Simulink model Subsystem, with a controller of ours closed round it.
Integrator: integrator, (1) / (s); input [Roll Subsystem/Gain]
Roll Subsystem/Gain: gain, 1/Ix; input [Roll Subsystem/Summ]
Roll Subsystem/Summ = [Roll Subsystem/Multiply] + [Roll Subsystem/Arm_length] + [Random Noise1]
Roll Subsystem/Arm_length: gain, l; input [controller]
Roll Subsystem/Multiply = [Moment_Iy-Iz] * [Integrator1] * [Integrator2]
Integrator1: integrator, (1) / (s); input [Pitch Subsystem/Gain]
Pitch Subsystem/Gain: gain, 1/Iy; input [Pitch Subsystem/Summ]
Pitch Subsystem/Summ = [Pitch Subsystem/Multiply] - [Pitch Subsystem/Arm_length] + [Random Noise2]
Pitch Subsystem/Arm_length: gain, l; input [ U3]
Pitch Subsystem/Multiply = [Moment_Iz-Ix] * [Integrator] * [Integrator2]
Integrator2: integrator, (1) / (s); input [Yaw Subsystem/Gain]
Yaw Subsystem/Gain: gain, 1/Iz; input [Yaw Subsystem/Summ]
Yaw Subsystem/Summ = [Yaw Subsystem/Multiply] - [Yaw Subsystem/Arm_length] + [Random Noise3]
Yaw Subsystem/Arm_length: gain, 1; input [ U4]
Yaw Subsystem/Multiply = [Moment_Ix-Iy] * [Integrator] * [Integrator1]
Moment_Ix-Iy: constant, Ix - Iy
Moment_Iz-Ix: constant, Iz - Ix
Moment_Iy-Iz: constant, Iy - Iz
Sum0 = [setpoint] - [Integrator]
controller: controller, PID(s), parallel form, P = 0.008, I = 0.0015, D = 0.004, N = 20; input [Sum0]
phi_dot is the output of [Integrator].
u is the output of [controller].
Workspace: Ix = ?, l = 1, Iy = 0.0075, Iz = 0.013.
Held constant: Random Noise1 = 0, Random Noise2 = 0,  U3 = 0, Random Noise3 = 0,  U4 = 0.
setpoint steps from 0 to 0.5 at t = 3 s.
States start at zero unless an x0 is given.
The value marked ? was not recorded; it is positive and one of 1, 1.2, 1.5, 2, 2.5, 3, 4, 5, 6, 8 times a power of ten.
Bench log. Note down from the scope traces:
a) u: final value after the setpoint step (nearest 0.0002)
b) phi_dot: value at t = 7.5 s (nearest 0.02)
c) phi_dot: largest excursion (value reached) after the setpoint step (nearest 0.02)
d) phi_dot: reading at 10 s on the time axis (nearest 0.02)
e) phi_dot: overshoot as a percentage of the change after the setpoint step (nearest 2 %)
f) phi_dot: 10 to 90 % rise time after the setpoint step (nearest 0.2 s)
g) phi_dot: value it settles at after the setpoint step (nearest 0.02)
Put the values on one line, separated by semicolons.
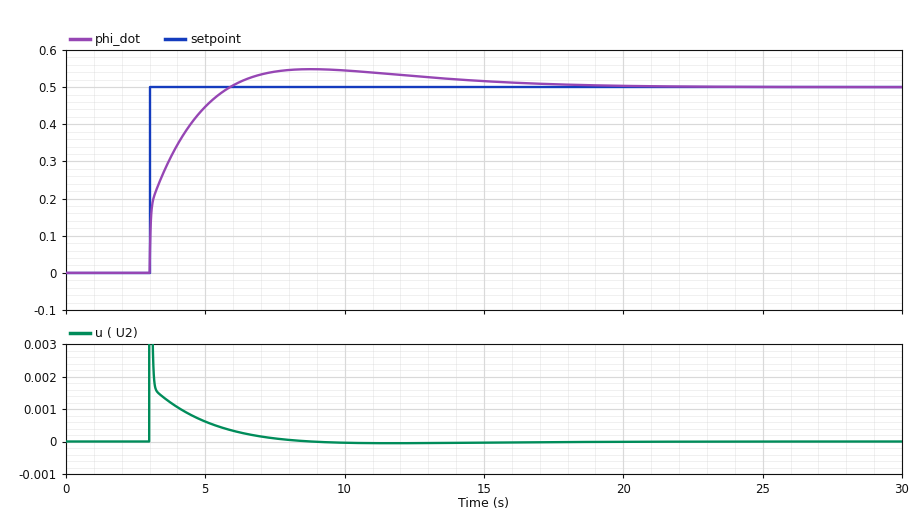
0.0000; 0.54; 0.54; 0.54; 10 %; 2.0 s; 0.50
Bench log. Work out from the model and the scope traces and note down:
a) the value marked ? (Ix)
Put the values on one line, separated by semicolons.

0.008
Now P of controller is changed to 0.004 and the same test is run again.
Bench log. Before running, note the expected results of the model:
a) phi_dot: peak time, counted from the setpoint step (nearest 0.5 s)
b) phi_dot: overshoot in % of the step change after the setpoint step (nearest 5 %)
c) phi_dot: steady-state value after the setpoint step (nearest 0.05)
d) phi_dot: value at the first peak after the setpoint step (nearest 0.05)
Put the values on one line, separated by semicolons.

7.0 s; 20 %; 0.50; 0.60
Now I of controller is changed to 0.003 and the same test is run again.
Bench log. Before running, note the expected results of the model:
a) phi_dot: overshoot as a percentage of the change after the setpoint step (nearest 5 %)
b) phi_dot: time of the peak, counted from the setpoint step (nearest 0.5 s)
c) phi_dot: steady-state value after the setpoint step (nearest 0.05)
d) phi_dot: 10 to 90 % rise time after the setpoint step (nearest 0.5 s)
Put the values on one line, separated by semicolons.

15 %; 4.5 s; 0.50; 1.5 s
